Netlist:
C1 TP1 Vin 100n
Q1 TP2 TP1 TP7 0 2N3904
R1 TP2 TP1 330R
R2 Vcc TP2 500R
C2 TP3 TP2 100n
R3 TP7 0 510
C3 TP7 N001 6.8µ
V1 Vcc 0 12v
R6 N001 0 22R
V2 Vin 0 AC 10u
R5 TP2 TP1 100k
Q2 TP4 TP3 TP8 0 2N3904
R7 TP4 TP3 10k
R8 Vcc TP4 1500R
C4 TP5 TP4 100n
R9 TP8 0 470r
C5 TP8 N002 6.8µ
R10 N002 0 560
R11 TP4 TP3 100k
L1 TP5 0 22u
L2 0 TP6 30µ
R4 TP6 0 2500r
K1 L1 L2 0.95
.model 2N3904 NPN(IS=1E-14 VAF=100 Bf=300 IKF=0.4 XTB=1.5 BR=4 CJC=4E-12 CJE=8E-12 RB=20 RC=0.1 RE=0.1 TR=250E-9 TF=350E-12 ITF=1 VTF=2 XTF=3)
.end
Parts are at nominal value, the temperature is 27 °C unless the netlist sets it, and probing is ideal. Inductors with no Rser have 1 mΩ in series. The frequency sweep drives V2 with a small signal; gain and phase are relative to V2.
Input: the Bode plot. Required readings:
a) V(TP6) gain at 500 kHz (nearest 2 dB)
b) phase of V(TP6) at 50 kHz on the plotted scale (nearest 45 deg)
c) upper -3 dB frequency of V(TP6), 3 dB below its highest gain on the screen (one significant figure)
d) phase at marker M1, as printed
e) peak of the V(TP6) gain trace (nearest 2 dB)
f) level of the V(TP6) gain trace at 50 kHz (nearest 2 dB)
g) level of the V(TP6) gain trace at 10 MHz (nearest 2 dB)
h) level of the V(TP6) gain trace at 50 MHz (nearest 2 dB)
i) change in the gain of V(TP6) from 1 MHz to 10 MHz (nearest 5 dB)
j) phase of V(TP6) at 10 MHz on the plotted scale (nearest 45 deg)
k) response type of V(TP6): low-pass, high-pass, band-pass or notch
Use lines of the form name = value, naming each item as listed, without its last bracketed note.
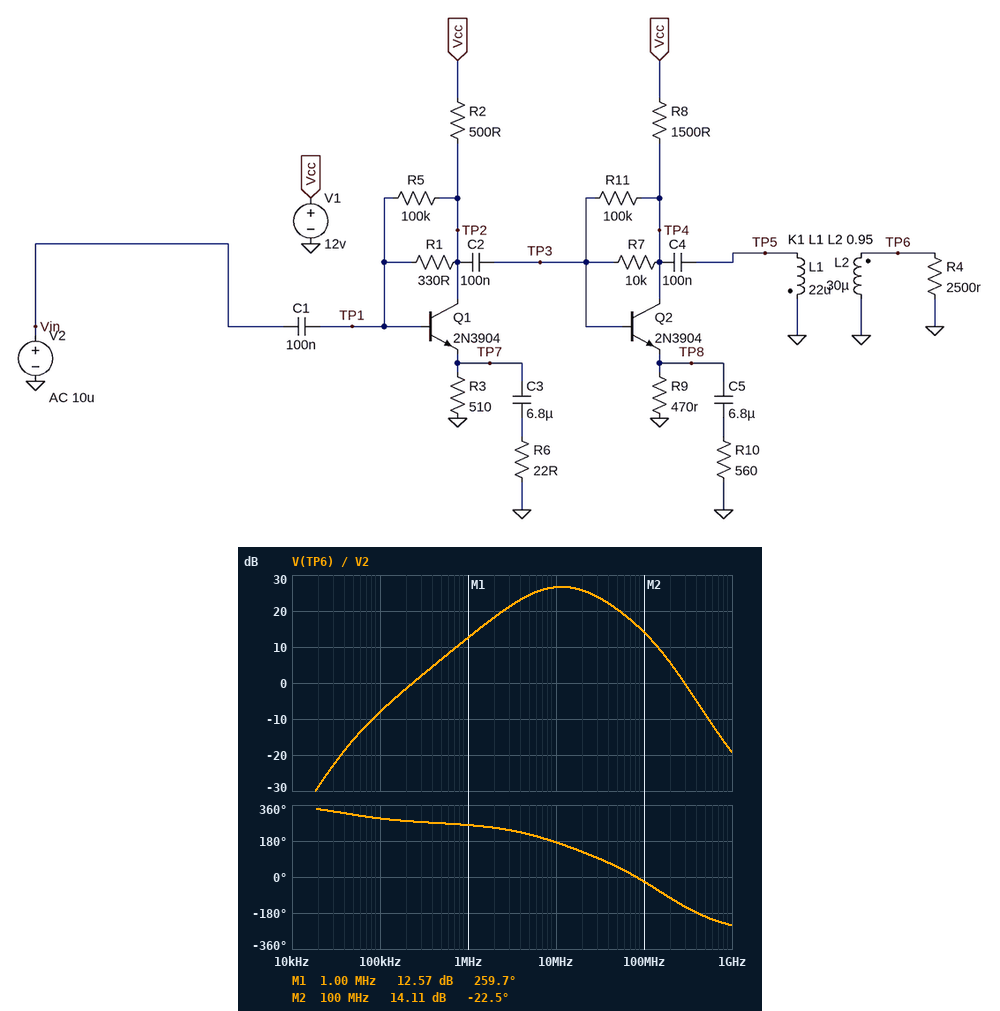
V(TP6) gain at 500 kHz = 6 dB
phase of V(TP6) at 50 kHz on the plotted scale = 315 deg
upper -3 dB frequency of V(TP6), 3 dB below its highest gain on the screen = 30 MHz
phase at marker M1, as printed = 259.7 deg
peak of the V(TP6) gain trace = 26 dB
level of the V(TP6) gain trace at 50 kHz = -16 dB
level of the V(TP6) gain trace at 10 MHz = 26 dB
level of the V(TP6) gain trace at 50 MHz = 20 dB
change in the gain of V(TP6) from 1 MHz to 10 MHz = 15 dB
phase of V(TP6) at 10 MHz on the plotted scale = 180 deg
response type of V(TP6): low-pass, high-pass, band-pass or notch = band-pass
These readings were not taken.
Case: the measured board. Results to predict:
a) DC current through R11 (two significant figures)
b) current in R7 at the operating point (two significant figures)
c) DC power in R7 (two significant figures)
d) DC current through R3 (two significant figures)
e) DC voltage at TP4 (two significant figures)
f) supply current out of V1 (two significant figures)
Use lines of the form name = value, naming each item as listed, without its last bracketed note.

DC current through R11 = 1.7 µA
current in R7 at the operating point = 17 µA
DC power in R7 = 3.0 µW
DC current through R3 = 11 mA
DC voltage at TP4 = 3.5 V
supply current out of V1 = 17 mA
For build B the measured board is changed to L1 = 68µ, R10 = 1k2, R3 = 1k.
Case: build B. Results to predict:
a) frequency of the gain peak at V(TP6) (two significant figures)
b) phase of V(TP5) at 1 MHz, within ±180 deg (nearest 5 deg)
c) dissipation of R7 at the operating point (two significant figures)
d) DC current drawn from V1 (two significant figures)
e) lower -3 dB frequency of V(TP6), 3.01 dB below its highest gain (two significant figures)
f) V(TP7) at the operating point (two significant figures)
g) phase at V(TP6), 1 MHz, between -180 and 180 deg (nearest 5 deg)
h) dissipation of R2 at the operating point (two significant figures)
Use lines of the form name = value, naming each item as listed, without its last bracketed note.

frequency of the gain peak at V(TP6) = 7.2 MHz
phase of V(TP5) at 1 MHz, within ±180 deg = 65 deg
dissipation of R7 at the operating point = 3.0 µW
DC current drawn from V1 = 13 mA
lower -3 dB frequency of V(TP6), 3.01 dB below its highest gain = 2.1 MHz
V(TP7) at the operating point = 7.5 V
phase at V(TP6), 1 MHz, between -180 and 180 deg = -115 deg
dissipation of R2 at the operating point = 28 mW
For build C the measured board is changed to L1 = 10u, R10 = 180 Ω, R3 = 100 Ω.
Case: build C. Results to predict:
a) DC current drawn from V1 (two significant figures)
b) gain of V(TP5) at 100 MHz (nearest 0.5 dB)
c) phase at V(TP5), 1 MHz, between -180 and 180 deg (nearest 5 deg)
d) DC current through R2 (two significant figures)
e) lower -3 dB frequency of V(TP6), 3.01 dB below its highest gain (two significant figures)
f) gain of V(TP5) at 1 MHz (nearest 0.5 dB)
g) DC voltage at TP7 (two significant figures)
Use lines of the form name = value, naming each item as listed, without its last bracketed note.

DC current drawn from V1 = 24 mA
gain of V(TP5) at 100 MHz = 18.0 dB
phase at V(TP5), 1 MHz, between -180 and 180 deg = 85 deg
DC current through R2 = 19 mA
lower -3 dB frequency of V(TP6), 3.01 dB below its highest gain = 5.7 MHz
gain of V(TP5) at 1 MHz = 12.5 dB
DC voltage at TP7 = 1.9 V
